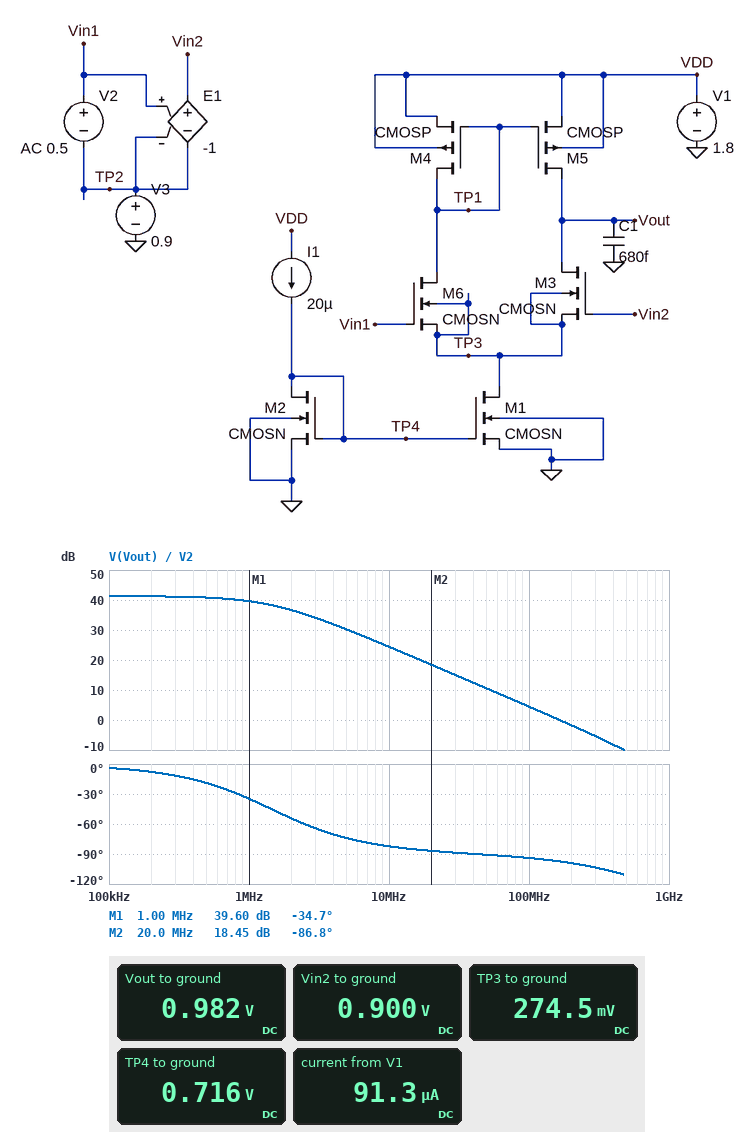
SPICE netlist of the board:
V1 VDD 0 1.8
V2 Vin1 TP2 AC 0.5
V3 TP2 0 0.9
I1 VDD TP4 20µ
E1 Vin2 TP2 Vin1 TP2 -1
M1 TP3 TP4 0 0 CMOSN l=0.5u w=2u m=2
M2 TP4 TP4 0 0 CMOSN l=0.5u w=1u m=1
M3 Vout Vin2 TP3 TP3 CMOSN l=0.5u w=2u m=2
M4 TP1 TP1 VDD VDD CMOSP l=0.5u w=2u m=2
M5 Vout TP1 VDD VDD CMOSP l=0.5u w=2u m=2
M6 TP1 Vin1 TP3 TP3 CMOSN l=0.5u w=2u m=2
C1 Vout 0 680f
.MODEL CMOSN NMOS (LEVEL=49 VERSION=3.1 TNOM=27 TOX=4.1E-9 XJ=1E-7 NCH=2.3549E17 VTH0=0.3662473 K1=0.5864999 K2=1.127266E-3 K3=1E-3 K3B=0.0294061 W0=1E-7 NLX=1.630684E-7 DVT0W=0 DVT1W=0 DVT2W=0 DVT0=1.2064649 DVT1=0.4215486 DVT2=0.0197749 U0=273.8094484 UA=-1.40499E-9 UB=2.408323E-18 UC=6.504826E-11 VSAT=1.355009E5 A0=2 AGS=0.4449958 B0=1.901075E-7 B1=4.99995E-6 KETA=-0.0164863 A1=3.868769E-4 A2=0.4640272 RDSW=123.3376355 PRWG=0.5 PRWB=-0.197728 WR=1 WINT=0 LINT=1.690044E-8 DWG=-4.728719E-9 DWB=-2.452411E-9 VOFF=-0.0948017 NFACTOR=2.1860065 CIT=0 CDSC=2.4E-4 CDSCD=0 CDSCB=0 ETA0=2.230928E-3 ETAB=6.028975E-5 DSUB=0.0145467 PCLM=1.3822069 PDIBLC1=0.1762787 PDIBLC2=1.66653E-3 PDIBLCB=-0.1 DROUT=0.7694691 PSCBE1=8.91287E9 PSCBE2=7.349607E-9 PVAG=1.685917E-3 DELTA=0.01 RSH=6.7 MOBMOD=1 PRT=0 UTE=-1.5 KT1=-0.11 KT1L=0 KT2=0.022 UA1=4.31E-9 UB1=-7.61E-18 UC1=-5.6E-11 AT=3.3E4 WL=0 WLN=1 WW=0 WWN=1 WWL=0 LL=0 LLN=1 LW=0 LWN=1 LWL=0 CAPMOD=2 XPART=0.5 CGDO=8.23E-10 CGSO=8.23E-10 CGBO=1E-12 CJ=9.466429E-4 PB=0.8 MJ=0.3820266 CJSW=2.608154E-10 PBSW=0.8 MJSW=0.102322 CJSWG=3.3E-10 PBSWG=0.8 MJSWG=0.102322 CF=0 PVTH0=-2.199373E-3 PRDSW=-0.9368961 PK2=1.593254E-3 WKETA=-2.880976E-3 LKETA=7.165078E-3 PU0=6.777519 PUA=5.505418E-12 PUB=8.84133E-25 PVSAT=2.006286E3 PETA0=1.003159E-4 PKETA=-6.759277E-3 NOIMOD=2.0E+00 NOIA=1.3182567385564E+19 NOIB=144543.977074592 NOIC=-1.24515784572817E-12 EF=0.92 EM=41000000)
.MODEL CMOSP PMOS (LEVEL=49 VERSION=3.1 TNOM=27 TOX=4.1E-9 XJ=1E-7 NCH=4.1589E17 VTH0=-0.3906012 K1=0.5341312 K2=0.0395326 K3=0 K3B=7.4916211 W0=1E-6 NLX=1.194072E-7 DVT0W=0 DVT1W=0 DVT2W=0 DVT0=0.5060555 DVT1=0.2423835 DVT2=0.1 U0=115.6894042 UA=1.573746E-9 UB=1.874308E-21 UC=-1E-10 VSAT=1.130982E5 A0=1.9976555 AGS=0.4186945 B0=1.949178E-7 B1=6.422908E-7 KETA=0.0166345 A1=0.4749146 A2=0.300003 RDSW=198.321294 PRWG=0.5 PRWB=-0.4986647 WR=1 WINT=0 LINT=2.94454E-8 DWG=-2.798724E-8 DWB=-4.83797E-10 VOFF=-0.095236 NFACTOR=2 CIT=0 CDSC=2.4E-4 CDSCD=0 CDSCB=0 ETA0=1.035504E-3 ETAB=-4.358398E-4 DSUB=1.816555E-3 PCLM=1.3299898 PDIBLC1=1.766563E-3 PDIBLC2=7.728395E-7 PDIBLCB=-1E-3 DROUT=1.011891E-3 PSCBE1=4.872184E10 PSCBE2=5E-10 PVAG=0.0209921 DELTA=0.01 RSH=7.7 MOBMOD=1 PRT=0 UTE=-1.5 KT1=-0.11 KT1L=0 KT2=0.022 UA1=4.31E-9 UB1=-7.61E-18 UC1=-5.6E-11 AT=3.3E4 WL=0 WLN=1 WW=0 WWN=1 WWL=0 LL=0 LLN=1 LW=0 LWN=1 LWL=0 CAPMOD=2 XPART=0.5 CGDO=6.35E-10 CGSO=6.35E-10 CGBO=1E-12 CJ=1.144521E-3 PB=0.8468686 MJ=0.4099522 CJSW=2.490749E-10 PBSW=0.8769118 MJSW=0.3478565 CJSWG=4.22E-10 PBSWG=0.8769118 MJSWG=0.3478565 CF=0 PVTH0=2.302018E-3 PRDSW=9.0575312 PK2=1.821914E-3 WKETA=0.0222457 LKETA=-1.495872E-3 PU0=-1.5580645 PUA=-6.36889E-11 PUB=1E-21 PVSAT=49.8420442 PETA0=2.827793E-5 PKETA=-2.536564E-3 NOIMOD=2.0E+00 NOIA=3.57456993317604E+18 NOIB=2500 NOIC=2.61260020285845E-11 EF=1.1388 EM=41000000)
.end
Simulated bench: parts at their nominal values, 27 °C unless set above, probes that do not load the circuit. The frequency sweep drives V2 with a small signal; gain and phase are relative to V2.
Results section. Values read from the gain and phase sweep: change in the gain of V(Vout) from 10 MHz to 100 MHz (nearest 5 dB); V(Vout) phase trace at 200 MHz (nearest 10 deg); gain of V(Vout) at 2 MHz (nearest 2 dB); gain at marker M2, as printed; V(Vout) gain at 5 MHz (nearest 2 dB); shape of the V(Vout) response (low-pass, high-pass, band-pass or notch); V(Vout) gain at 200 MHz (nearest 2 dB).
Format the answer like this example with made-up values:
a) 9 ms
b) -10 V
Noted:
a) -20 dB
b) -100 deg
c) 36 dB
d) 18.45 dB
e) 30 dB
f) low-pass
g) -2 dB
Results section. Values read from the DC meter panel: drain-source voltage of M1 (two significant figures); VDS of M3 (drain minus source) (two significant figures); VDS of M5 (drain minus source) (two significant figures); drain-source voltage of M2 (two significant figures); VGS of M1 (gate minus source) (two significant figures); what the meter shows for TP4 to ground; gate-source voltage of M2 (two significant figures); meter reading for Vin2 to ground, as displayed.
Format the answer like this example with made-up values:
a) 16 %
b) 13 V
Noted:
a) 270 mV
b) 710 mV
c) -820 mV
d) 720 mV
e) 720 mV
f) 0.716 V
g) 720 mV
h) 0.900 V
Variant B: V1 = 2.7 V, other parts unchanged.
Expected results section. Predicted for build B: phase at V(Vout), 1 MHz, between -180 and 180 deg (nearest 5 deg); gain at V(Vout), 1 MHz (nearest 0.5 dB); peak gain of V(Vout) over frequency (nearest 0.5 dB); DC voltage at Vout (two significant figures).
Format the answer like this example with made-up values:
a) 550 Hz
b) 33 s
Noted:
a) -40 deg
b) 40.5 dB
c) 42.5 dB
d) 1.9 V
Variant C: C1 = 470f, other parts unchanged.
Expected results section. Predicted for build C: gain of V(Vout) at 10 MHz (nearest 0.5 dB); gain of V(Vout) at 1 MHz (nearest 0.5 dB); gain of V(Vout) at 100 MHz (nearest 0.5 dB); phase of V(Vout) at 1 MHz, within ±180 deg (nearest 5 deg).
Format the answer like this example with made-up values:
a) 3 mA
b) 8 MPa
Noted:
a) 27.5 dB
b) 40.5 dB
c) 7.5 dB
d) -25 deg
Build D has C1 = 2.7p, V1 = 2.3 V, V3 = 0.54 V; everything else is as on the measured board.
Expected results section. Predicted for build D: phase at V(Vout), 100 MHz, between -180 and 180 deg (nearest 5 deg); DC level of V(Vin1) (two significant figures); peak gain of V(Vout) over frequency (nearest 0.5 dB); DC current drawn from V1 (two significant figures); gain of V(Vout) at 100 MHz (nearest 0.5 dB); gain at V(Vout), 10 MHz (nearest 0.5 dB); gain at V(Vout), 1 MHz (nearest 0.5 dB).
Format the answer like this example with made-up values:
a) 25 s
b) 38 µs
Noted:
a) -100 deg
b) 540 mV
c) 43.0 dB
d) 36 µA
e) -15.5 dB
f) 4.5 dB
g) 24.5 dB
